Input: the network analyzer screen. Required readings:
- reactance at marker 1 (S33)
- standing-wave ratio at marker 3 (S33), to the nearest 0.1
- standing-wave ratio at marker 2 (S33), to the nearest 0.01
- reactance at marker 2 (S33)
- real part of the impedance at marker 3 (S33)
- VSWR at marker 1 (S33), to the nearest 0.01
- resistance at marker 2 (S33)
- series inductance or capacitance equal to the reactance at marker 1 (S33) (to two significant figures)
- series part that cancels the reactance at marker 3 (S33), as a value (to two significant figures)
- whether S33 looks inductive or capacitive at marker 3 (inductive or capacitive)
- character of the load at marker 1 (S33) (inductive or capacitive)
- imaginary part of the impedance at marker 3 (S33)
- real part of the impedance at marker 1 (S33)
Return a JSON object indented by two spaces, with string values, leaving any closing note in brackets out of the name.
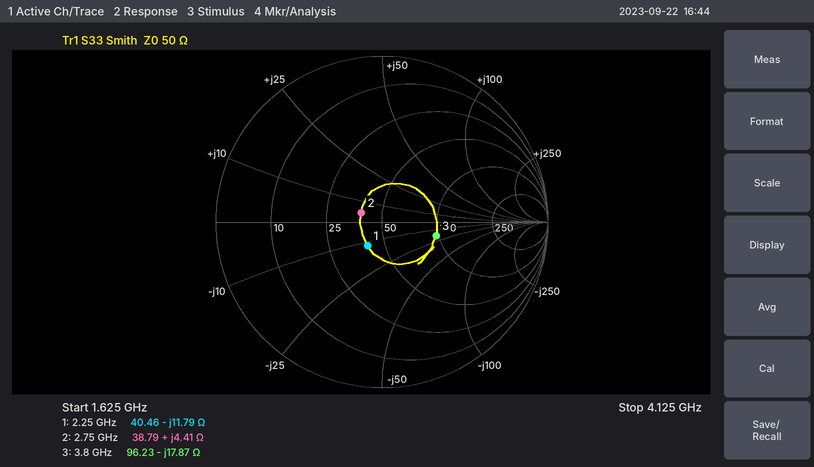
{
  "reactance at marker 1": "-11.79 Ω",
  "standing-wave ratio at marker 3 (S33), to the nearest 0.1": "2.0",
  "standing-wave ratio at marker 2 (S33), to the nearest 0.01": "1.31",
  "reactance at marker 2": "+4.41 Ω",
  "real part of the impedance at marker 3": "96.23 Ω",
  "VSWR at marker 1 (S33), to the nearest 0.01": "1.40",
  "resistance at marker 2": "38.79 Ω",
  "series inductance or capacitance equal to the reactance at marker 1 (S33)": "6.0 pF",
  "series part that cancels the reactance at marker 3 (S33), as a value": "750 pH",
  "whether S33 looks inductive or capacitive at marker 3": "capacitive",
  "character of the load at marker 1 (S33)": "capacitive",
  "imaginary part of the impedance at marker 3": "-17.87 Ω",
  "real part of the impedance at marker 1": "40.46 Ω"
}
